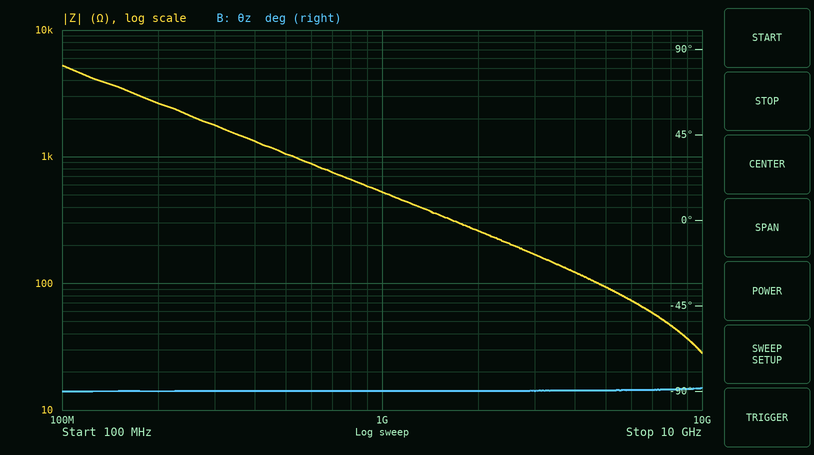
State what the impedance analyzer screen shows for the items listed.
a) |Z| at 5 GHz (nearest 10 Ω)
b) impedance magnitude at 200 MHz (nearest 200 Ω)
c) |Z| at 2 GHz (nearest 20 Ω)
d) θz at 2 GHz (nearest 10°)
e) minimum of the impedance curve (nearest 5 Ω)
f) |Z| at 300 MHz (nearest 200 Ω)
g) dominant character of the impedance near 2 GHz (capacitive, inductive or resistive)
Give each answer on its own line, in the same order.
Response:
90 Ω
2.6 kΩ
260 Ω
-90°
30 Ω
1.8 kΩ
capacitive
